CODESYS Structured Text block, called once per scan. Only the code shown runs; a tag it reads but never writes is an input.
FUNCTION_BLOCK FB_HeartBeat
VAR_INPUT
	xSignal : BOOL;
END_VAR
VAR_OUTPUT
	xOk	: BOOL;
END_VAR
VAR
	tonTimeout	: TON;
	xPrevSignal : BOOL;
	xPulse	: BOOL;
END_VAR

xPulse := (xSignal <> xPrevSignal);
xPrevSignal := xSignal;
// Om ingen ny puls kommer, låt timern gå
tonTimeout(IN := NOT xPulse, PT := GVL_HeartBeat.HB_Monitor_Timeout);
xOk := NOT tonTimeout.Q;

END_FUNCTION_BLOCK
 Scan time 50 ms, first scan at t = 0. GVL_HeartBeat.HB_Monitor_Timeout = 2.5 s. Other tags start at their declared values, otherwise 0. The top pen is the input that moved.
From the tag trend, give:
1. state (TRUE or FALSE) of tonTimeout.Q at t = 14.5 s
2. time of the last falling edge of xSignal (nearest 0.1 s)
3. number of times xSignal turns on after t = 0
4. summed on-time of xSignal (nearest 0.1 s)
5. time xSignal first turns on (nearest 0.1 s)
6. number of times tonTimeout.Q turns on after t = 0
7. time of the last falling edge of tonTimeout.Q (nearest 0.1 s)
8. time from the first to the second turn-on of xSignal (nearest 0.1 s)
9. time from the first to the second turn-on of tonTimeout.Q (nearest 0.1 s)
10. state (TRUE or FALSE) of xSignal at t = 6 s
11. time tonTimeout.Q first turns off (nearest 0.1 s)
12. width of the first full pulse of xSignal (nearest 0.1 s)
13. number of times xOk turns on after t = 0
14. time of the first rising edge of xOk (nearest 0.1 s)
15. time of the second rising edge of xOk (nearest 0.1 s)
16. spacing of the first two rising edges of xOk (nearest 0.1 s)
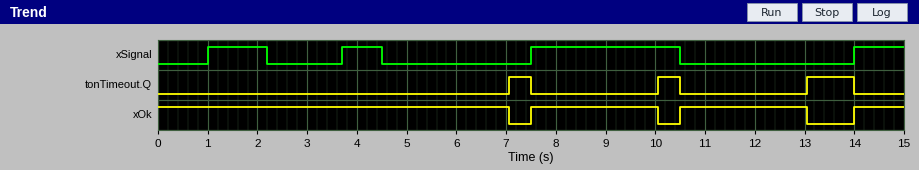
FALSE
10.5 s
4
6.0 s
1.0 s
3
14.0 s
2.7 s
3.0 s
FALSE
7.5 s
1.2 s
3
7.5 s
10.5 s
3.0 s
